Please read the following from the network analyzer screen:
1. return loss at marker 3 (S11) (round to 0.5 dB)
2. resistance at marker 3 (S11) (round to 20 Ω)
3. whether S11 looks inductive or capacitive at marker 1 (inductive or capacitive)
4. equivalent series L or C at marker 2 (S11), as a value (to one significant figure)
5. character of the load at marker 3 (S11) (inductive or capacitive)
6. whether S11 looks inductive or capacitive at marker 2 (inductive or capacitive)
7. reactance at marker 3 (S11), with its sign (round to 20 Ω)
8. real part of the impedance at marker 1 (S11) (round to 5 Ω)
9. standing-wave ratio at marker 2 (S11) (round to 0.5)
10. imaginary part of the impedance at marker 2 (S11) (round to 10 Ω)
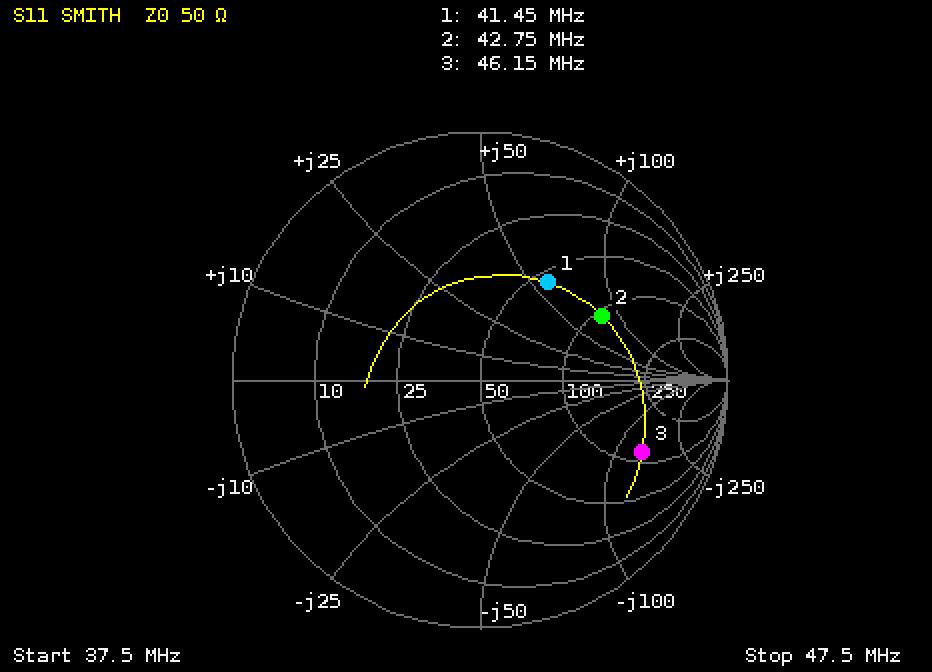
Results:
3.0 dB
120 Ω
inductive
300 nH
capacitive
inductive
-140 Ω
55 Ω
3.5
+80 Ω
